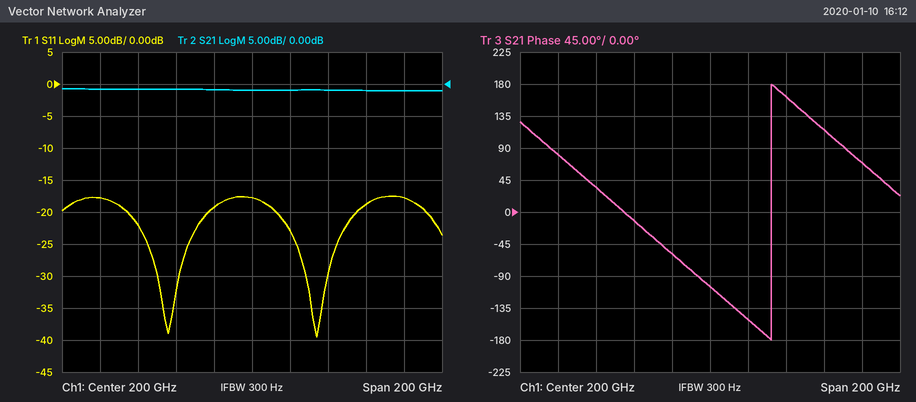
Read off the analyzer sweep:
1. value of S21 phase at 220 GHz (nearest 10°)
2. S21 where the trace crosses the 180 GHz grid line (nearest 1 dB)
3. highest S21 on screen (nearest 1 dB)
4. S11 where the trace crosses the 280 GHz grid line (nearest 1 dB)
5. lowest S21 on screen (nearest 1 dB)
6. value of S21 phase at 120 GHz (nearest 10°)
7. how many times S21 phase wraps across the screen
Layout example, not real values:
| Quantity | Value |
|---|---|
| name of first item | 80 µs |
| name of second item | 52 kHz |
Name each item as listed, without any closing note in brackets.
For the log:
| Quantity | Value |
|---|---|
| value of S21 phase at 220 GHz | -150° |
| S21 where the trace crosses the 180 GHz grid line | -1 dB |
| highest S21 on screen | -1 dB |
| S11 where the trace crosses the 280 GHz grid line | -18 dB |
| lowest S21 on screen | -1 dB |
| value of S21 phase at 120 GHz | 80° |
| how many times S21 phase wraps across the screen | 1 |
